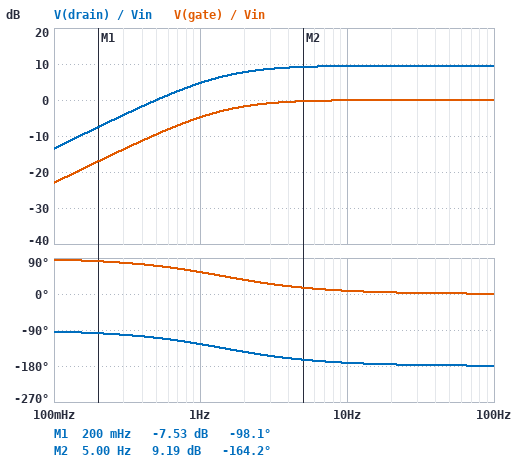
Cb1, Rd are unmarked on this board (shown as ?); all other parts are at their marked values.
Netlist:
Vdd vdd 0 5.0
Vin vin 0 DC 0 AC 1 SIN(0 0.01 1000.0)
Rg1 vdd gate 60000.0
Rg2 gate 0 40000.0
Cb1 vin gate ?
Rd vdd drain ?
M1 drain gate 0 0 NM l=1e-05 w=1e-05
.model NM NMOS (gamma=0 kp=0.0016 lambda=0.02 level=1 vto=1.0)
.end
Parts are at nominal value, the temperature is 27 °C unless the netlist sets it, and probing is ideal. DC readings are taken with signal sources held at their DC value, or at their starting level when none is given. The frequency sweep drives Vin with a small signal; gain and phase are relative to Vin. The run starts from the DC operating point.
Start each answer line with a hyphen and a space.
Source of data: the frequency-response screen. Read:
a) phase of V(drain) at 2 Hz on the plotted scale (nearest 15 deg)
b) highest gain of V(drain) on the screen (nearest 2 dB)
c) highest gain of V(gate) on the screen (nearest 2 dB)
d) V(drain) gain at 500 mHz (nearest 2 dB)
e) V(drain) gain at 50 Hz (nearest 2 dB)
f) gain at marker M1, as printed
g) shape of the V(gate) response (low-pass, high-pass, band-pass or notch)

- -150 deg
- 10 dB
- 0 dB
- 0 dB
- 10 dB
- -7.53 dB
- high-pass
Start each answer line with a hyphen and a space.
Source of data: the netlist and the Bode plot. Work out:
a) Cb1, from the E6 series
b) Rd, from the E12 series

- 4.7 µF
- 1.8 kΩ
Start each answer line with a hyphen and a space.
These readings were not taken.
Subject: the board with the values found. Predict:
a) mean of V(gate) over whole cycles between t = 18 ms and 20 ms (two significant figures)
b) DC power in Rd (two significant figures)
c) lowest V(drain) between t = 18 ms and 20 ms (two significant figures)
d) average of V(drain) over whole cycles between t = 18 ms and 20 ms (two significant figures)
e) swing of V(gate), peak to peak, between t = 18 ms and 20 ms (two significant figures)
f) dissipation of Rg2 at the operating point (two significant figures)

- 2.0 V
- 1.3 mW
- 3.4 V
- 3.5 V
- 20 mV
- 100 µW
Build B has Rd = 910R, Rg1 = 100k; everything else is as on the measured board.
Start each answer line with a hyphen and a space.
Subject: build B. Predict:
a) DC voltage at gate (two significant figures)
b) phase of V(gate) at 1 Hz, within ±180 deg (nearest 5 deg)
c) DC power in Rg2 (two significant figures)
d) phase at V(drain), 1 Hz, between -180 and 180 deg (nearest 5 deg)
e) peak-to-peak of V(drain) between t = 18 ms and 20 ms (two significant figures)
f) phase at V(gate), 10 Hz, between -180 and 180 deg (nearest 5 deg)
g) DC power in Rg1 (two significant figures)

- 1.4 V
- 50 deg
- 51 µW
- -130 deg
- 14 mV
- 5 deg
- 130 µW
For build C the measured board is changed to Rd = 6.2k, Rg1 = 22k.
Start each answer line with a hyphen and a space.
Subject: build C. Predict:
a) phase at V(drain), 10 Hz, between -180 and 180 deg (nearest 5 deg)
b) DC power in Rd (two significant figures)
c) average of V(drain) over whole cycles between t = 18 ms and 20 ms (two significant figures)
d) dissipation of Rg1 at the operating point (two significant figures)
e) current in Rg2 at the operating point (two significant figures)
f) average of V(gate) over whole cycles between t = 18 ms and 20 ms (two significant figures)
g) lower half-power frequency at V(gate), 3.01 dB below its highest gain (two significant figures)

- -165 deg
- 3.7 mW
- 230 mV
- 140 µW
- 81 µA
- 3.2 V
- 2.4 Hz
